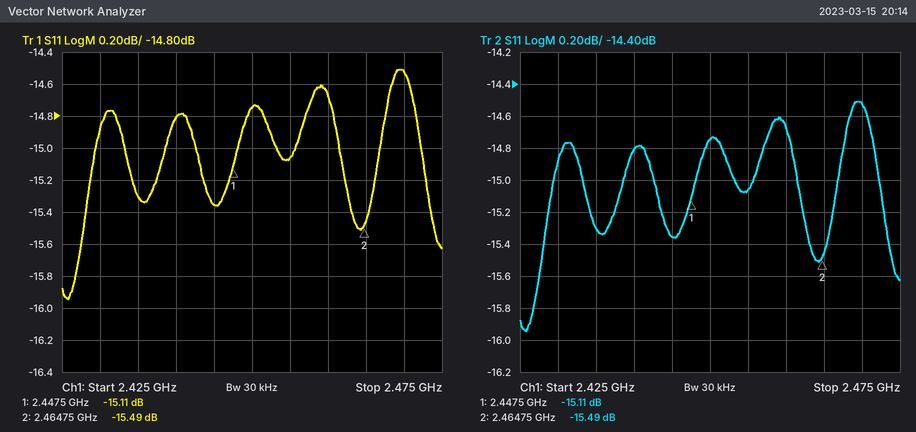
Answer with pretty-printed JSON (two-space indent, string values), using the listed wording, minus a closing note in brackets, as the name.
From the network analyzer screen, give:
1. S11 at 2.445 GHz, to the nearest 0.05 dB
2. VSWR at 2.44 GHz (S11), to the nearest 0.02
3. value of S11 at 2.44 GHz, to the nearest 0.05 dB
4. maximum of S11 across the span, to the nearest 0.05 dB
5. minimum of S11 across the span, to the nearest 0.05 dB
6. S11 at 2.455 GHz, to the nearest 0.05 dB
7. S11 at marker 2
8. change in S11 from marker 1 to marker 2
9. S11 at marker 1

{
  "S11 at 2.445 GHz, to the nearest 0.05 dB": "-15.35 dB",
  "VSWR at 2.44 GHz (S11), to the nearest 0.02": "1.44",
  "value of S11 at 2.44 GHz, to the nearest 0.05 dB": "-14.80 dB",
  "maximum of S11 across the span, to the nearest 0.05 dB": "-14.50 dB",
  "minimum of S11 across the span, to the nearest 0.05 dB": "-15.95 dB",
  "S11 at 2.455 GHz, to the nearest 0.05 dB": "-15.05 dB",
  "S11 at marker 2": "-15.49 dB",
  "change in S11 from marker 1 to marker 2": "-0.38 dB",
  "S11 at marker 1": "-15.11 dB"
}
